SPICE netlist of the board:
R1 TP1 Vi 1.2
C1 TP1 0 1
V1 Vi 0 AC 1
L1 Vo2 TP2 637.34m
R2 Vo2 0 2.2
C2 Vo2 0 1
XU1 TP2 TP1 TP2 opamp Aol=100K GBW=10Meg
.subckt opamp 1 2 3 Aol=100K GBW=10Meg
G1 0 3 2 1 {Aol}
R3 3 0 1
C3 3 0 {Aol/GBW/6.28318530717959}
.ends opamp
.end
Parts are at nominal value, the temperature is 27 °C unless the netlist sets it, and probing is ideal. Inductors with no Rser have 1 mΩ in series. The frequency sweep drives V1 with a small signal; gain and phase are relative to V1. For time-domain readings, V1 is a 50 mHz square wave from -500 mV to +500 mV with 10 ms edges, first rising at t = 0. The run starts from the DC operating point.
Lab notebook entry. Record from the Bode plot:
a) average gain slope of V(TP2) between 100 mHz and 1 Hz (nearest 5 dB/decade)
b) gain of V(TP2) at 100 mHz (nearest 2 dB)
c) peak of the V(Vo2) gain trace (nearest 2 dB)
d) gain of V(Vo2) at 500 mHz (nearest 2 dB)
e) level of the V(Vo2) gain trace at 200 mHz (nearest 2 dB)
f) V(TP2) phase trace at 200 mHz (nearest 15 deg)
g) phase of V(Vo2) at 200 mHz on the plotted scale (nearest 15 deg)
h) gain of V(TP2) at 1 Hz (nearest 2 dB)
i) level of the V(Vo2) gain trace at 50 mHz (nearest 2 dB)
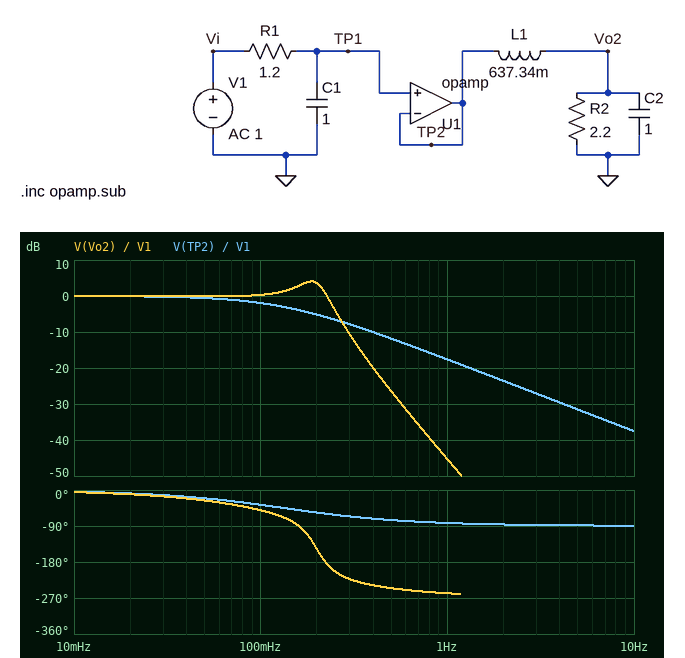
-15 dB/decade
-2 dB
4 dB
-26 dB
4 dB
-60 deg
-150 deg
-18 dB
0 dB
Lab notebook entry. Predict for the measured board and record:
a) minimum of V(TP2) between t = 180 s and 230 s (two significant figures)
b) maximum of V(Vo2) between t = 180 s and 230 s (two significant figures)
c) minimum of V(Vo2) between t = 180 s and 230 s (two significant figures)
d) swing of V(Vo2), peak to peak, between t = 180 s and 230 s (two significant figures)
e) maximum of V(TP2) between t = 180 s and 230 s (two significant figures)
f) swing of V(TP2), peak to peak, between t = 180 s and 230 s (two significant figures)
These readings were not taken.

-500 mV
710 mV
-710 mV
1.4 V
500 mV
1.0 V
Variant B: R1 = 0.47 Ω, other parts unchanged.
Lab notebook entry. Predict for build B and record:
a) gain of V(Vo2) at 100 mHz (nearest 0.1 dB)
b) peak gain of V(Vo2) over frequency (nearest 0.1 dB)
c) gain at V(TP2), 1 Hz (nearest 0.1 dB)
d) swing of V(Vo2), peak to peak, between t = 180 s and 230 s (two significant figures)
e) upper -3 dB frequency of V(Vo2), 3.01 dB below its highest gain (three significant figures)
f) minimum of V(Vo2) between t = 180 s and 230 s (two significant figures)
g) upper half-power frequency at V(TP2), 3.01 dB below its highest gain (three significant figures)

1.9 dB
7.7 dB
-9.9 dB
1.9 V
224 mHz
-930 mV
339 mHz
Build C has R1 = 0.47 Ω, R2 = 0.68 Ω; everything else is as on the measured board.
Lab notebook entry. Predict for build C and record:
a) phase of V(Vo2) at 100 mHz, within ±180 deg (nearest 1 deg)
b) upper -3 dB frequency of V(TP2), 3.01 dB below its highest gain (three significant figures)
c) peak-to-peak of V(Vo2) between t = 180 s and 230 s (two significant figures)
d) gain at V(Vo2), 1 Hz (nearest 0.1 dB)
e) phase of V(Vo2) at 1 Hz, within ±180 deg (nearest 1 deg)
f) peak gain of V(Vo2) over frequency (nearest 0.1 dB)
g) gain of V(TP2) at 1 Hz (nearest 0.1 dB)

-55 deg
339 mHz
1.2 V
-37.8 dB
122 deg
0.1 dB
-9.9 dB
